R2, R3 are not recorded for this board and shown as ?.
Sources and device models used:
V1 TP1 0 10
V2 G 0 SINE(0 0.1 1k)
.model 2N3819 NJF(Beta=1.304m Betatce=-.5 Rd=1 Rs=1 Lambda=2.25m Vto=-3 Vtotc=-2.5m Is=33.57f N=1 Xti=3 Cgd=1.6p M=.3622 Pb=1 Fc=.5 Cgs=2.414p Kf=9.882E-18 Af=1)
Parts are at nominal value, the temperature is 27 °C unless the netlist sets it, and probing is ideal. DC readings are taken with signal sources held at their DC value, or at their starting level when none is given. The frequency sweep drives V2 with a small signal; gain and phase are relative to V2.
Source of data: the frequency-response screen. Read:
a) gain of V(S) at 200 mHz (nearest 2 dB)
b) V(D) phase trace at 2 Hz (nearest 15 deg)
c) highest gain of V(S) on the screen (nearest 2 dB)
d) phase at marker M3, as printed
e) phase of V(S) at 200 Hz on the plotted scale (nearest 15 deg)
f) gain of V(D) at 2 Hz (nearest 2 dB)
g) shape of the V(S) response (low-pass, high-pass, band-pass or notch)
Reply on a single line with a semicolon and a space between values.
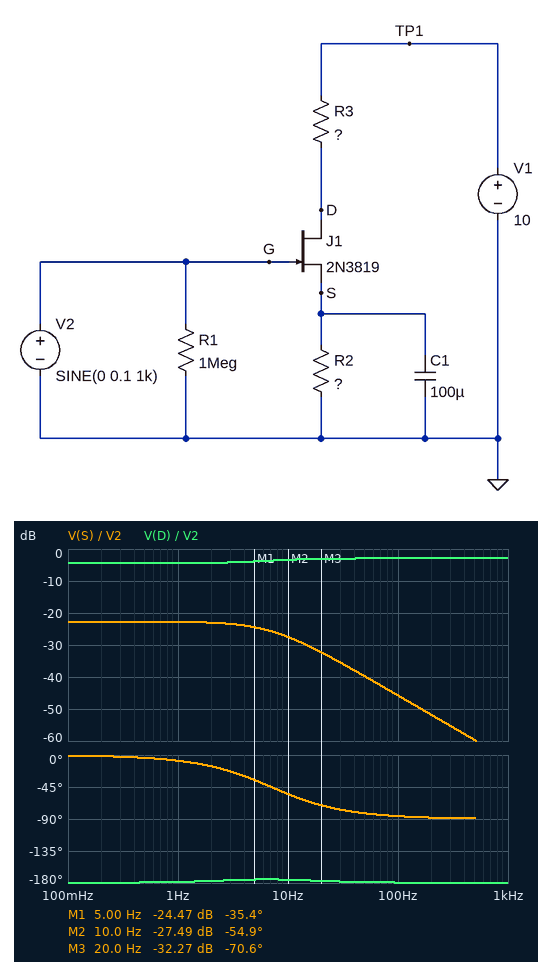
-22 dB; -180 deg; -22 dB; -70.6 deg; -90 deg; -4 dB; low-pass
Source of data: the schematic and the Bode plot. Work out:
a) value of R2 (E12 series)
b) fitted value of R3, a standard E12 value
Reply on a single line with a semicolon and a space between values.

270 Ω; 2.2 kΩ
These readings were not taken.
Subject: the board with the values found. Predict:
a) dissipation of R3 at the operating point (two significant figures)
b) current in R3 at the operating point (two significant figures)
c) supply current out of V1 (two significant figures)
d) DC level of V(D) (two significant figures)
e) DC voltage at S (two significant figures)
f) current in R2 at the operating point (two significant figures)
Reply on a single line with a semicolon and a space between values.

30 mW; 3.7 mA; 3.7 mA; 1.9 V; 990 mV; 3.7 mA
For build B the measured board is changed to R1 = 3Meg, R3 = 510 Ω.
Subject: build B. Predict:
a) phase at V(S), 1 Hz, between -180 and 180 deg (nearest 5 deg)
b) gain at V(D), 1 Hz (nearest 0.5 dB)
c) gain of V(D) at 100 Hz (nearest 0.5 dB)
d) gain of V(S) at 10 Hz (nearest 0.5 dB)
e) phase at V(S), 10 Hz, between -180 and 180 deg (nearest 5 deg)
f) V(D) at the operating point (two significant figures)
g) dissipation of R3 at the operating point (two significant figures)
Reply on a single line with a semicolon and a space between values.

-5 deg; 0.5 dB; 7.5 dB; -7.0 dB; -35 deg; 7.8 V; 9.7 mW
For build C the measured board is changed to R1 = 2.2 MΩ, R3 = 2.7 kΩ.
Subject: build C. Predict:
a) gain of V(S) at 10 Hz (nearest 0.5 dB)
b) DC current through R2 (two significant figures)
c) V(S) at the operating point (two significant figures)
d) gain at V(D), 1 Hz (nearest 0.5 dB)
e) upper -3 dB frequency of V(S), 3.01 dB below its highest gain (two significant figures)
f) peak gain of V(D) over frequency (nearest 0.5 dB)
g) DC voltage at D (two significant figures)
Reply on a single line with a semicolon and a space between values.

-34.0 dB; 3.1 mA; 850 mV; -9.0 dB; 6.7 Hz; -8.0 dB; 1.5 V
